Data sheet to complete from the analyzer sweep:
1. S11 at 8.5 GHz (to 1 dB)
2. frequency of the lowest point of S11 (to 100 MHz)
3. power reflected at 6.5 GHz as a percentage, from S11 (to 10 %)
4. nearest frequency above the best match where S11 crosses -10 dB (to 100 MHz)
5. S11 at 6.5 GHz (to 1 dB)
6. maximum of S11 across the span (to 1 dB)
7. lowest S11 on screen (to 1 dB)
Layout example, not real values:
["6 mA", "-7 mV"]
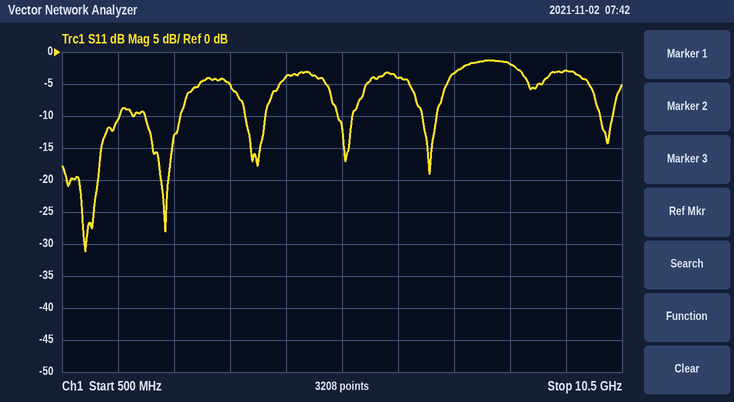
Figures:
["-2 dB", "900 MHz", "40 %", "1.5 GHz", "-4 dB", "-1 dB", "-31 dB"]
